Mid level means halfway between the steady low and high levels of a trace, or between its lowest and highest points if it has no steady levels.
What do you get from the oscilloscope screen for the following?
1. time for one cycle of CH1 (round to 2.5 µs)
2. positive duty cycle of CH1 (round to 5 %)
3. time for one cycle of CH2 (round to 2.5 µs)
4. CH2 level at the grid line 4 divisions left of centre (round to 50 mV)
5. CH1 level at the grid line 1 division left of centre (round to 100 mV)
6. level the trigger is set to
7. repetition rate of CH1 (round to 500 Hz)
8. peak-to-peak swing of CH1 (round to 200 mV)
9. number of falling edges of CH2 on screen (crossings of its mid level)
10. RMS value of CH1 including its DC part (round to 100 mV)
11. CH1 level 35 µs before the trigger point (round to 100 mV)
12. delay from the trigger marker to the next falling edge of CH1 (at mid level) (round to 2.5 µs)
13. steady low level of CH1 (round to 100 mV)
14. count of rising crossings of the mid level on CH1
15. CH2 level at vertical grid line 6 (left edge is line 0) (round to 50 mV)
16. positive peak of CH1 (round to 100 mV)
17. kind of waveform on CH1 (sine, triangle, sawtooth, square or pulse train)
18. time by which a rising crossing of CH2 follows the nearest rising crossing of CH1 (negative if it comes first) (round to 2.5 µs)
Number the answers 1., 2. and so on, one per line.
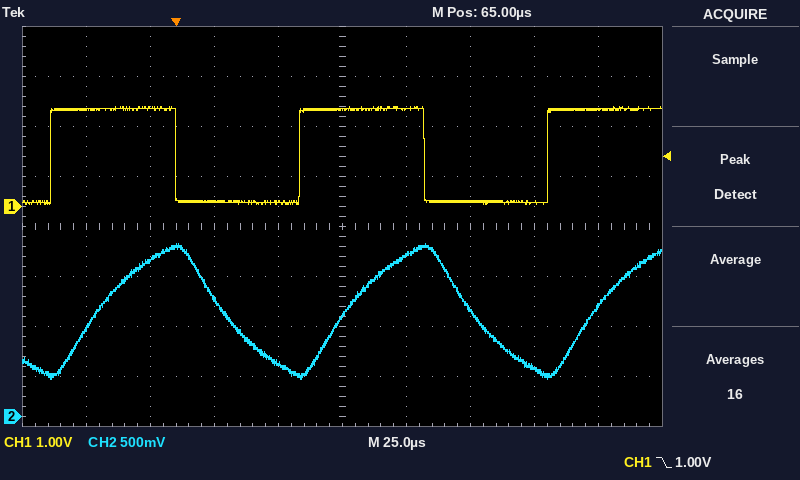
1. 97.5 µs
2. 50 %
3. 97.5 µs
4. 900 mV
5. 100 mV
6. 1.00 V
7. 10.5 kHz
8. 2.0 V
9. 2
10. 1.4 V
11. 1.9 V
12. 97.5 µs
13. 100 mV
14. 3
15. 1.60 V
16. 2.0 V
17. square
18. +17.5 µs
